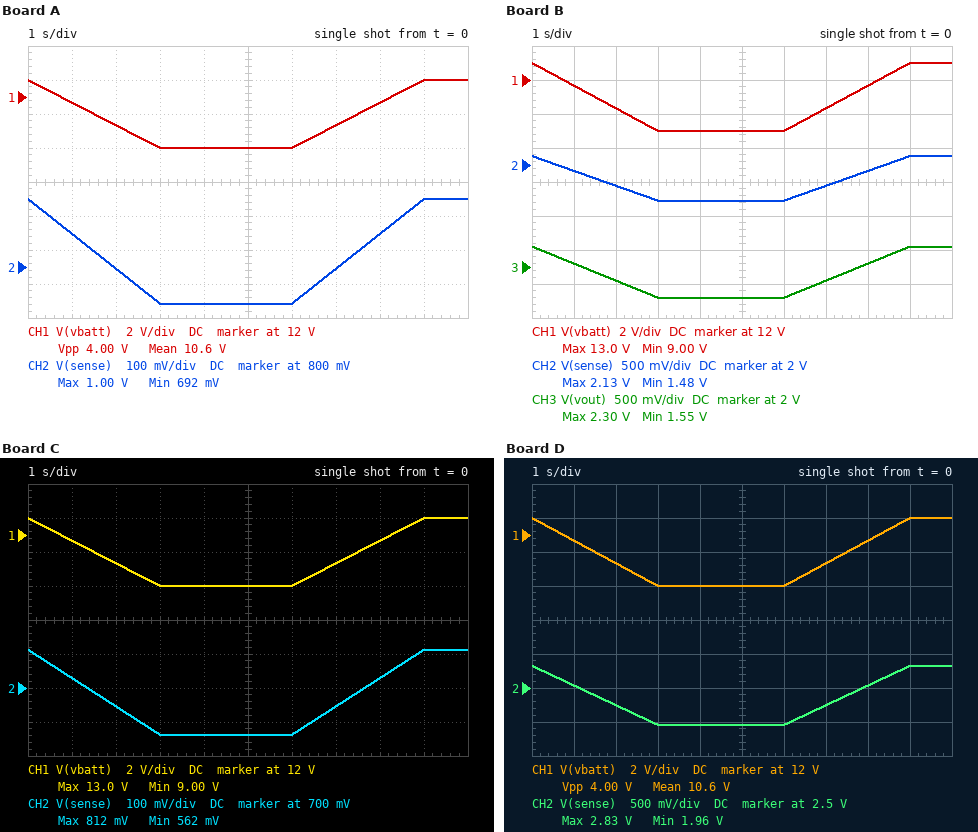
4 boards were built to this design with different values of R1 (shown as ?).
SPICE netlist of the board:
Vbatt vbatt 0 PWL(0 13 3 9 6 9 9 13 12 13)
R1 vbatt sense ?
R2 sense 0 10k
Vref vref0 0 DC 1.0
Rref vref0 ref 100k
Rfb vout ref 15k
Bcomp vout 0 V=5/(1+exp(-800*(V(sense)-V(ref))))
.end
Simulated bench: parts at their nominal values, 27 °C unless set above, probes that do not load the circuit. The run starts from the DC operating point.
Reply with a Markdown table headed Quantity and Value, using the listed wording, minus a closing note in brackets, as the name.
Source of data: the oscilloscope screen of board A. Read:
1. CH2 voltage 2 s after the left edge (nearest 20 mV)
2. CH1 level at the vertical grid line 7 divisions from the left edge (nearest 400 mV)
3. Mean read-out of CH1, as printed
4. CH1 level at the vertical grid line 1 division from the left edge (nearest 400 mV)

| Quantity | Value |
|---|---|
| CH2 voltage 2 s after the left edge | 800 mV |
| CH1 level at the vertical grid line 7 divisions from the left edge | 10.4 V |
| Mean read-out of CH1, as printed | 10.6 V |
| CH1 level at the vertical grid line 1 division from the left edge | 11.6 V |
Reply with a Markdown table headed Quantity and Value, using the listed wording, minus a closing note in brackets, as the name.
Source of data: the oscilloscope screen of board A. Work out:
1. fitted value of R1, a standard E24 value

| Quantity | Value |
|---|---|
| fitted value of R1, a standard E24 value | 120 kΩ |
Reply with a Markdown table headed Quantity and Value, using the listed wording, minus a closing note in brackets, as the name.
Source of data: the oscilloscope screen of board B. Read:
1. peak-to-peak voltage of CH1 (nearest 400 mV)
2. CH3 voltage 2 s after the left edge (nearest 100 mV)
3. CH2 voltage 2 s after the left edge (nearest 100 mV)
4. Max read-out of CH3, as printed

| Quantity | Value |
|---|---|
| peak-to-peak voltage of CH1 | 4.0 V |
| CH3 voltage 2 s after the left edge | 1.8 V |
| CH2 voltage 2 s after the left edge | 1.7 V |
| Max read-out of CH3, as printed | 2.30 V |
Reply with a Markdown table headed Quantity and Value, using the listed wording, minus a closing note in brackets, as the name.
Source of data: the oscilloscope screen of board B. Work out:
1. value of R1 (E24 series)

| Quantity | Value |
|---|---|
| value of R1 | 51 kΩ |
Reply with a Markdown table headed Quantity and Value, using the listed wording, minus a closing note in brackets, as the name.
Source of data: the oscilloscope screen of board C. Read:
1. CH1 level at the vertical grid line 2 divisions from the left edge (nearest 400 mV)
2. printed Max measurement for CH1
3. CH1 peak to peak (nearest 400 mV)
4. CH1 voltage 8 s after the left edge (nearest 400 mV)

| Quantity | Value |
|---|---|
| CH1 level at the vertical grid line 2 divisions from the left edge | 10.4 V |
| printed Max measurement for CH1 | 13.0 V |
| CH1 peak to peak | 4.0 V |
| CH1 voltage 8 s after the left edge | 11.6 V |
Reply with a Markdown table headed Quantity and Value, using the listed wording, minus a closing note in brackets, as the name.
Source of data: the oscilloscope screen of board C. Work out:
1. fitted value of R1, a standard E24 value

| Quantity | Value |
|---|---|
| fitted value of R1, a standard E24 value | 150 kΩ |
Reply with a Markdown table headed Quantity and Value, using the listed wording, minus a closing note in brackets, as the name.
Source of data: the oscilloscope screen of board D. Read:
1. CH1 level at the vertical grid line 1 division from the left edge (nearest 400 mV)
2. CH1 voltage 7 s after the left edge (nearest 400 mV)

| Quantity | Value |
|---|---|
| CH1 level at the vertical grid line 1 division from the left edge | 11.6 V |
| CH1 voltage 7 s after the left edge | 10.4 V |
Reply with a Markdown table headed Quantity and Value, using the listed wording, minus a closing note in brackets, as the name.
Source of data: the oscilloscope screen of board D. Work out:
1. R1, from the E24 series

| Quantity | Value |
|---|---|
| R1, from the E24 series | 36 kΩ |
